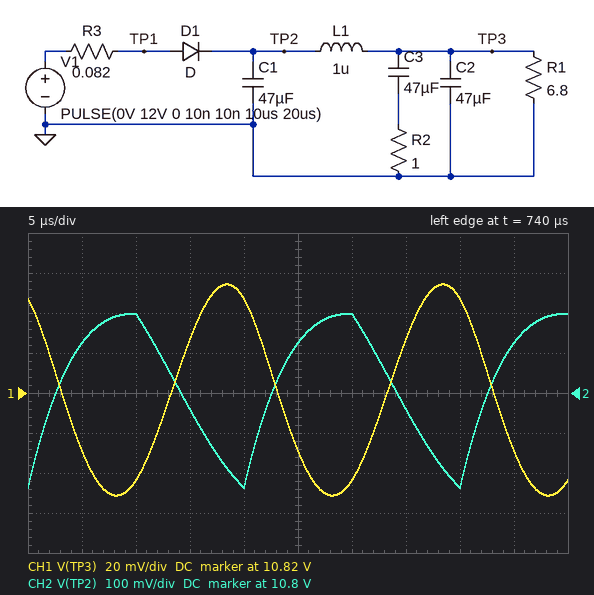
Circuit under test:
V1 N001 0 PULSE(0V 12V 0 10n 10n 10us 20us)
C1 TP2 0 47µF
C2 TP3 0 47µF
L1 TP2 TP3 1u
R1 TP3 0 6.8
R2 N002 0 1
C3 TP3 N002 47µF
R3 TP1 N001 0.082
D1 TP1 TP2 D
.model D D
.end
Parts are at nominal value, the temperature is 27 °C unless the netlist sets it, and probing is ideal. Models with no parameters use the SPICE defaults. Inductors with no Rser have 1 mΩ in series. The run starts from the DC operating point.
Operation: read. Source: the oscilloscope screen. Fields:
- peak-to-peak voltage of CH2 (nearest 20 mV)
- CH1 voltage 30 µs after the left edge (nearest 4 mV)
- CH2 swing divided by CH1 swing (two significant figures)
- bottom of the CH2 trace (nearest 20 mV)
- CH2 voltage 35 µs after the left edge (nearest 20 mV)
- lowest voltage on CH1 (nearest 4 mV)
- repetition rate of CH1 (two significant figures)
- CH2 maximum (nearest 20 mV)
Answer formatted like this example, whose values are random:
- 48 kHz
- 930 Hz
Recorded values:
- 440 mV
- 10.776 V
- 4.1
- 10.56 V
- 10.76 V
- 10.768 V
- 50 kHz
- 11.00 V
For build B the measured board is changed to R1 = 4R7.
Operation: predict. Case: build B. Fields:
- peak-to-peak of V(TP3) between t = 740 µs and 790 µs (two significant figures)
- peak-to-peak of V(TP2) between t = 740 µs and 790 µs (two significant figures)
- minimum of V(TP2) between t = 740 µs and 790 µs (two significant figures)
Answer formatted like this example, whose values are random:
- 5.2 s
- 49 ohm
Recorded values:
- 150 mV
- 620 mV
- 10 V
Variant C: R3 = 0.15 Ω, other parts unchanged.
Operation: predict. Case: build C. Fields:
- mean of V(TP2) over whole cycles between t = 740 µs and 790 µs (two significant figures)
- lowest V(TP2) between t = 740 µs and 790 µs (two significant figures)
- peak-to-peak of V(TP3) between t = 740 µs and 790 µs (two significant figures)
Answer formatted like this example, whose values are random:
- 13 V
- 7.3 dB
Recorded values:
- 11 V
- 10 V
- 100 mV
